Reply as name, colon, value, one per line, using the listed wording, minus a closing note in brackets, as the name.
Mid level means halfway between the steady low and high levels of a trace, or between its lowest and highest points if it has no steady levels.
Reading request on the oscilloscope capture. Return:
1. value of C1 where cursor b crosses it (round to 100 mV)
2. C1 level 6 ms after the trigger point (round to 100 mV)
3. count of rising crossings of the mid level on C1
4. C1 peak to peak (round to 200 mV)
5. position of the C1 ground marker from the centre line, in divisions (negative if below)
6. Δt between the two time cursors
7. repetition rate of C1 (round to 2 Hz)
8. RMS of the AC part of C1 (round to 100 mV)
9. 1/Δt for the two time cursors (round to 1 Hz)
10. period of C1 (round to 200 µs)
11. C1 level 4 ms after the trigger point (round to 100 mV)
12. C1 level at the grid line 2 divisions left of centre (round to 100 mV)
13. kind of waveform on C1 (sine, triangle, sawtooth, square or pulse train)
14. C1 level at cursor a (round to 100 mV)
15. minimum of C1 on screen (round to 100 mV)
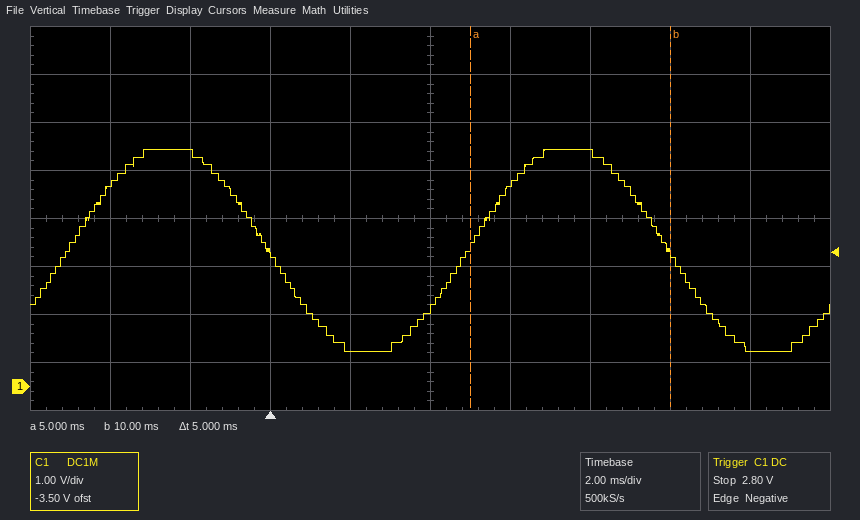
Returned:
value of C1 where cursor b crosses it: 2.8 V
C1 level 6 ms after the trigger point: 4.2 V
count of rising crossings of the mid level on C1: 2
C1 peak to peak: 4.2 V
position of the C1 ground marker from the centre line, in divisions: -3.5 div
Δt between the two time cursors: 5 ms
repetition rate of C1: 100 Hz
RMS of the AC part of C1: 1.5 V
1/Δt for the two time cursors: 200 Hz
period of C1: 10.0 ms
C1 level 4 ms after the trigger point: 1.6 V
C1 level at the grid line 2 divisions left of centre: 2.8 V
kind of waveform on C1: sine
C1 level at cursor a: 2.9 V
minimum of C1 on screen: 700 mV
